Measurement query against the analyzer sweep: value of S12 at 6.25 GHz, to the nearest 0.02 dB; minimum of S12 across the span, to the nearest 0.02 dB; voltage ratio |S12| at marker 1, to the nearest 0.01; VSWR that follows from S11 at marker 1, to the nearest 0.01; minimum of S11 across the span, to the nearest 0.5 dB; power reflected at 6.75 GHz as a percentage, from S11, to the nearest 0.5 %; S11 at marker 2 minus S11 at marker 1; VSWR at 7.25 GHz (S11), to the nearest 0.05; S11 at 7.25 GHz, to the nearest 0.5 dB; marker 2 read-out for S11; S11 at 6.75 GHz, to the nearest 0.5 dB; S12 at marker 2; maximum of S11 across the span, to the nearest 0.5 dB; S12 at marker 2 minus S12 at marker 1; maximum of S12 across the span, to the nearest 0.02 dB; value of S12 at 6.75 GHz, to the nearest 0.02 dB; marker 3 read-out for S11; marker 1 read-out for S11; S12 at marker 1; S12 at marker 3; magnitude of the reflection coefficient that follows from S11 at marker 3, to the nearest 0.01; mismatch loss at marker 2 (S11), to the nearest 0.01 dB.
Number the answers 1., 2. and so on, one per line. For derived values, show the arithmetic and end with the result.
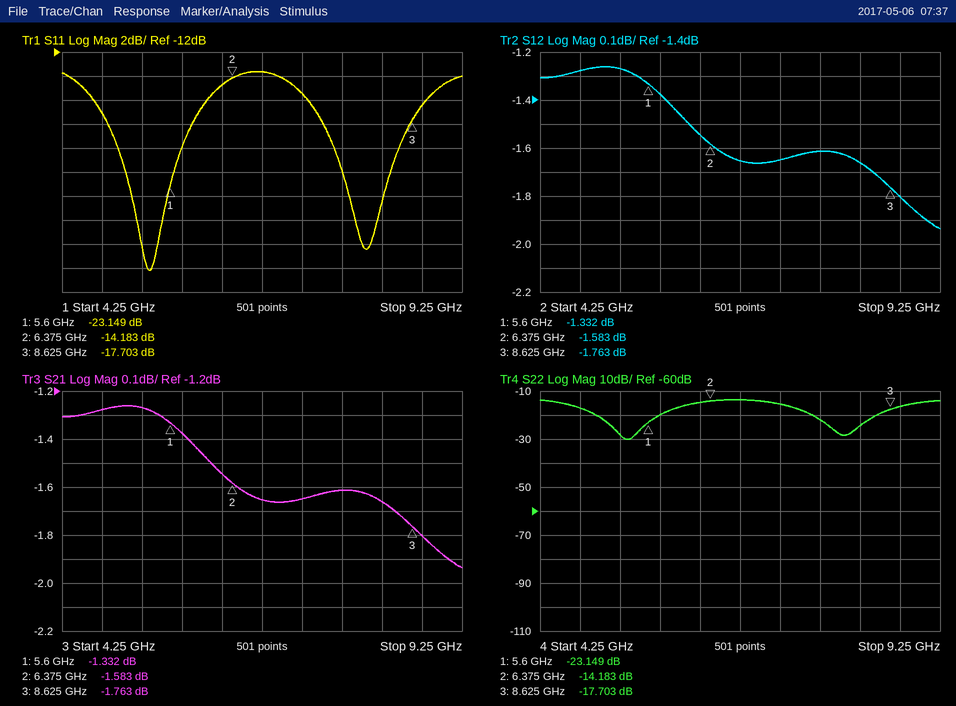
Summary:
1. -1.54 dB
2. -1.94 dB
3. 10^(-1.332/20) ≈ 0.86
4. (1 + 0.0696)/(1 − 0.0696) ≈ 1.15
5. -30.0 dB
6. 10^(-13.5/10) ≈ 4.5 %
7. -14.183 − (-23.149) = 8.966 dB
8. |Γ| = 10^(-15.5/20) = 0.1679; VSWR = (1 + 0.1679)/(1 − 0.1679) ≈ 1.40
9. -15.5 dB
10. -14.183 dB
11. -13.5 dB
12. -1.583 dB
13. -13.5 dB
14. -1.583 − (-1.332) = -0.251 dB
15. -1.26 dB
16. -1.66 dB
17. -17.703 dB
18. -23.149 dB
19. -1.332 dB
20. -1.763 dB
21. 10^(-17.703/20) ≈ 0.13
22. −10 log10(1 − 10^(-14.183/10)) ≈ 0.17 dB
